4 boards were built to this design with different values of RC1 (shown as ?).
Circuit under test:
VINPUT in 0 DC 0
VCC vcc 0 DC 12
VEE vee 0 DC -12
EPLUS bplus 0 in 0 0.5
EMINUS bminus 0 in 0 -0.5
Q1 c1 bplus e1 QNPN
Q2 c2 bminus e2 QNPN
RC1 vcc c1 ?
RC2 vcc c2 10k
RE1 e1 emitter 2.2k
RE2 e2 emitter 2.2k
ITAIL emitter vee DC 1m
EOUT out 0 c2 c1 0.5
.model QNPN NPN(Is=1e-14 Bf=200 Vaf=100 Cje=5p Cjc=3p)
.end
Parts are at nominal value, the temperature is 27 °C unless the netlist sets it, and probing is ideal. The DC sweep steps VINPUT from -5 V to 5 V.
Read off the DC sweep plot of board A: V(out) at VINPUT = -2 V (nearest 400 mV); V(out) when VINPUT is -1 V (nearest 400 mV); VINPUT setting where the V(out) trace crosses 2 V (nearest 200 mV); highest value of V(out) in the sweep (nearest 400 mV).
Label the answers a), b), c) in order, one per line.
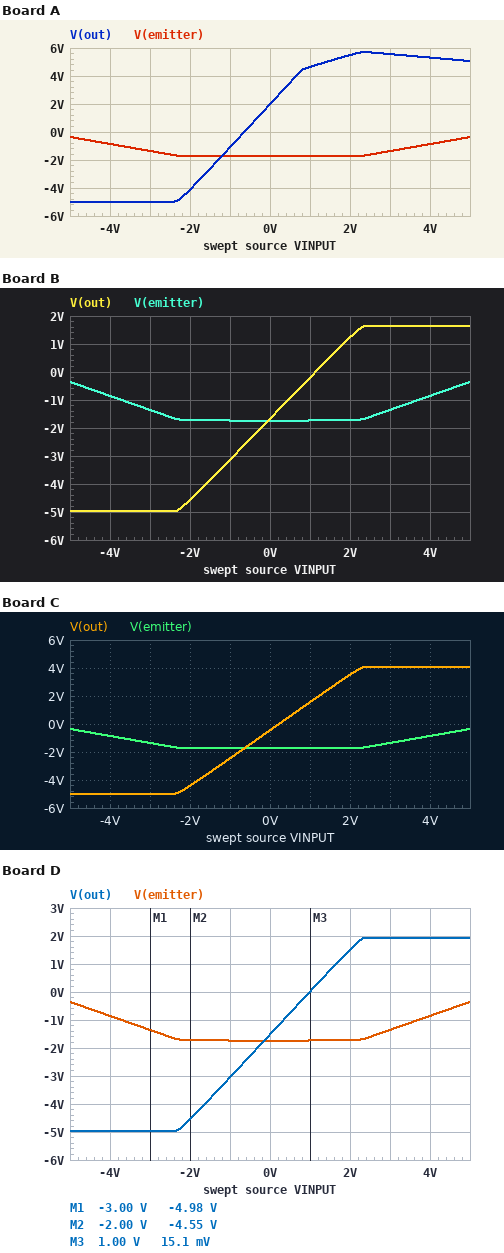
a) -4.0 V
b) -1.2 V
c) 0 V
d) 5.6 V
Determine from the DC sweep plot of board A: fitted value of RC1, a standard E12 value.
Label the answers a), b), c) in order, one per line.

a) 18 kΩ
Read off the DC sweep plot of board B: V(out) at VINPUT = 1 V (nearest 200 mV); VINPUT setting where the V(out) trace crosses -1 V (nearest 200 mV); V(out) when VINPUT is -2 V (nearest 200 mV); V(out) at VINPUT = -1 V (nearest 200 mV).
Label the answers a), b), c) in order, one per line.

a) -200 mV
b) 400 mV
c) -4.6 V
d) -3.2 V
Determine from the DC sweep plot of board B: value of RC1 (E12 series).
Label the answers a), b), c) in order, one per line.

a) 3.3 kΩ
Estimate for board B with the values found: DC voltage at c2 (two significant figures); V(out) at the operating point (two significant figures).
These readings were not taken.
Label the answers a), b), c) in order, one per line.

a) 7.0 V
b) -1.7 V
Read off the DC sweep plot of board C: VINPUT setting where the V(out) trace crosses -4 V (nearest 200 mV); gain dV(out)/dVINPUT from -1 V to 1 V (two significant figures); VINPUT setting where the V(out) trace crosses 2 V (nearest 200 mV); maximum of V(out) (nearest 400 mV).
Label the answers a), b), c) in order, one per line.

a) -1.8 V
b) 2.0 V/V
c) 1.2 V
d) 4.0 V
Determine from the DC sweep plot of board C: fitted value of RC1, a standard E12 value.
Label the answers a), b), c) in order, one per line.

a) 8.2 kΩ
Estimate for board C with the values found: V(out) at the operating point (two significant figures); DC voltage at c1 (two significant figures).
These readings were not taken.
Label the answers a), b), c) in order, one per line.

a) -450 mV
b) 7.9 V
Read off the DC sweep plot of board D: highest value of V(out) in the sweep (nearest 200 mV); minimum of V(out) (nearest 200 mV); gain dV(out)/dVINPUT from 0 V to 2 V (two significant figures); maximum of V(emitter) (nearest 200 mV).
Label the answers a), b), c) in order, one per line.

a) 2.0 V
b) -5.0 V
c) 1.5 V/V
d) -400 mV
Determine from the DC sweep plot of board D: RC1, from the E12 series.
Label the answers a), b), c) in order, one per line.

a) 3.9 kΩ
